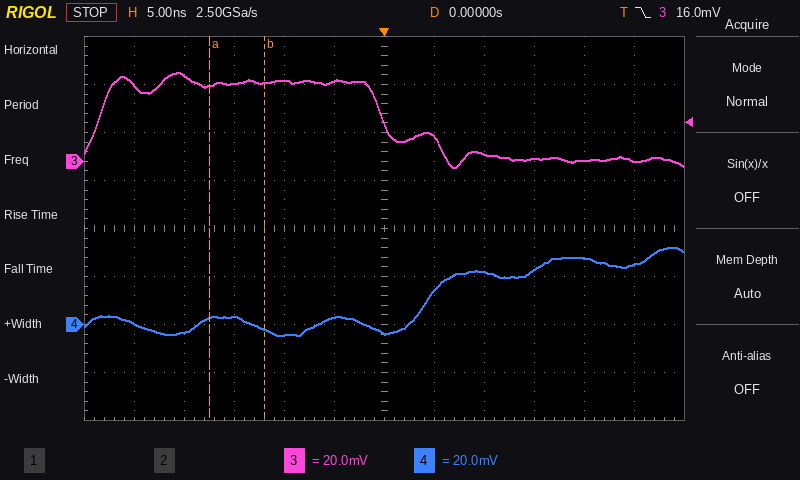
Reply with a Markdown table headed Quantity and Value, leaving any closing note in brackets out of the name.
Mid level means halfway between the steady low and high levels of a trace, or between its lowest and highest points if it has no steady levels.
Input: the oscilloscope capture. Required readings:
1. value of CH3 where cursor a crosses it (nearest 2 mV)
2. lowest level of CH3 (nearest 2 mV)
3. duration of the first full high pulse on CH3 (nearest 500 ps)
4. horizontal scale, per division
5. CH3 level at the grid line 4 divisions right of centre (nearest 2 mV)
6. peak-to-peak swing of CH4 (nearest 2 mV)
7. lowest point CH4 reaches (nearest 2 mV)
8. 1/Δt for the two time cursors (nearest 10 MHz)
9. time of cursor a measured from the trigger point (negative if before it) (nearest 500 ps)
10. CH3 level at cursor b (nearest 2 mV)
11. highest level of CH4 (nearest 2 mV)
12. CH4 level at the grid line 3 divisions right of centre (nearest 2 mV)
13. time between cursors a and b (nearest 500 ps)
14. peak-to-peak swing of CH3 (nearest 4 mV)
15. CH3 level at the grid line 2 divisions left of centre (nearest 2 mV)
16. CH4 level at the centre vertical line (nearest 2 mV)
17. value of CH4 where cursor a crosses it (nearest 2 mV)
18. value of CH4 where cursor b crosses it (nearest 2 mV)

| Quantity | Value |
|---|---|
| value of CH3 where cursor a crosses it | 32 mV |
| lowest level of CH3 | -2 mV |
| duration of the first full high pulse on CH3 | 28.5 ns |
| horizontal scale, per division | 5 ns |
| CH3 level at the grid line 4 divisions right of centre | 0 mV |
| peak-to-peak swing of CH4 | 36 mV |
| lowest point CH4 reaches | -4 mV |
| 1/Δt for the two time cursors | 180 MHz |
| time of cursor a measured from the trigger point (negative if before it) | -17.5 ns |
| CH3 level at cursor b | 32 mV |
| highest level of CH4 | 32 mV |
| CH4 level at the grid line 3 divisions right of centre | 22 mV |
| time between cursors a and b | 5.5 ns |
| peak-to-peak swing of CH3 | 40 mV |
| CH3 level at the grid line 2 divisions left of centre | 34 mV |
| CH4 level at the centre vertical line | -4 mV |
| value of CH4 where cursor a crosses it | 2 mV |
| value of CH4 where cursor b crosses it | -2 mV |
